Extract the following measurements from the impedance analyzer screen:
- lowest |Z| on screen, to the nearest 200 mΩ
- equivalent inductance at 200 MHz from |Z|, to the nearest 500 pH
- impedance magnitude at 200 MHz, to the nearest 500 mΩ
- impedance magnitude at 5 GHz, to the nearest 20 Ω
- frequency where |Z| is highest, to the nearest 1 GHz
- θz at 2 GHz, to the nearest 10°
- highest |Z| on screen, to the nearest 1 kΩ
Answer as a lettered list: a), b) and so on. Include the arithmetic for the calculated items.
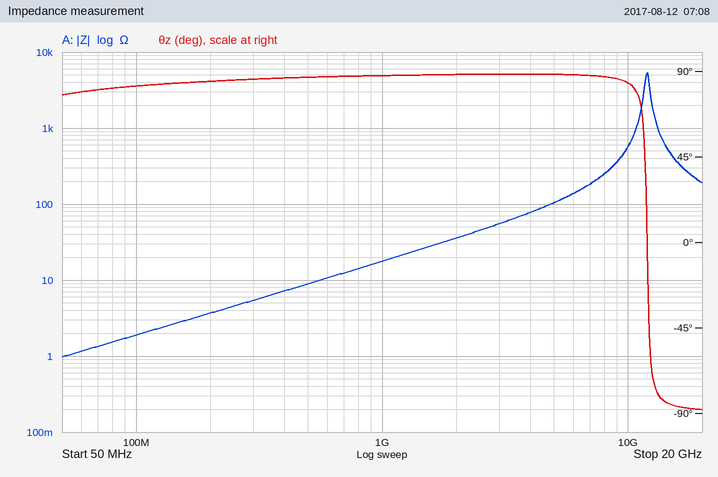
a) 1.0 Ω
b) L = 3.5 Ω/(2π × 200 MHz) ≈ 2.79 nH, so 3.0 nH to the nearest 500 pH
c) 3.5 Ω
d) 100 Ω
e) 12 GHz
f) 90°
g) 5 kΩ
